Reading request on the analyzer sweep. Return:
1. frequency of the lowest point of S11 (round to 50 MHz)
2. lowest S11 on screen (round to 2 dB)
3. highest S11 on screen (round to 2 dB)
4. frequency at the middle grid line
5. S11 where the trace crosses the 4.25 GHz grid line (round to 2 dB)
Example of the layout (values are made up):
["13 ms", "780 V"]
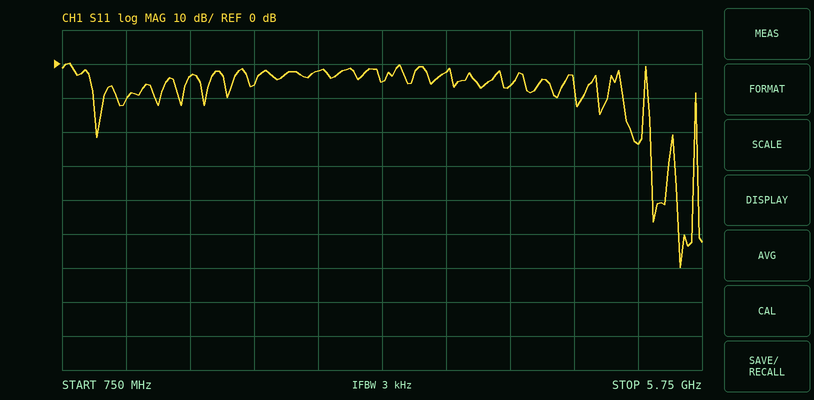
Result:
["5.60 GHz", "-60 dB", "0 dB", "3.25 GHz", "-6 dB"]
